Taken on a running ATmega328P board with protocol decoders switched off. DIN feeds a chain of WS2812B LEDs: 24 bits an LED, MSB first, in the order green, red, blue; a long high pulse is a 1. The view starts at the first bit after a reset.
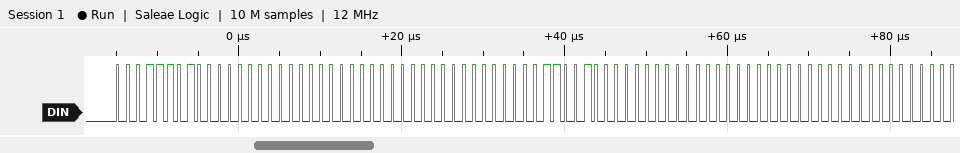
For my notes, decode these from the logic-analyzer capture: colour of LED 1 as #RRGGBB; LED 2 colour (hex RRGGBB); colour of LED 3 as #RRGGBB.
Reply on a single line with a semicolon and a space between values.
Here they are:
#001D00; #000032; #000000
